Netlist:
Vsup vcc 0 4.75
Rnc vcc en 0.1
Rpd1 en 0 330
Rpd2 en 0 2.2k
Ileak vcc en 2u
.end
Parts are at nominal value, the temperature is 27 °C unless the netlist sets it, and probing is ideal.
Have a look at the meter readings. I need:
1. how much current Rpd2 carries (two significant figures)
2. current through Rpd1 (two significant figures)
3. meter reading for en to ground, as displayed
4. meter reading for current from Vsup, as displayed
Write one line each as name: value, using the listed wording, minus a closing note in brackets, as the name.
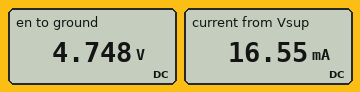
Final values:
how much current Rpd2 carries: 2.2 mA
current through Rpd1: 14 mA
meter reading for en to ground, as displayed: 4.748 V
meter reading for current from Vsup, as displayed: 16.55 mA
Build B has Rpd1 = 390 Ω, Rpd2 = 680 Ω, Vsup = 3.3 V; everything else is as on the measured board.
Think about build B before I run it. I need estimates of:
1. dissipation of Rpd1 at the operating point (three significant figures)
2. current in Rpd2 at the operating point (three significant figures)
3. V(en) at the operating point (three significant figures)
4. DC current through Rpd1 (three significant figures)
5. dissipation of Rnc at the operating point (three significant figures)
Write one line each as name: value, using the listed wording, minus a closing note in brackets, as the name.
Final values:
dissipation of Rpd1 at the operating point: 27.9 mW
current in Rpd2 at the operating point: 4.85 mA
V(en) at the operating point: 3.30 V
DC current through Rpd1: 8.46 mA
dissipation of Rnc at the operating point: 17.7 µW
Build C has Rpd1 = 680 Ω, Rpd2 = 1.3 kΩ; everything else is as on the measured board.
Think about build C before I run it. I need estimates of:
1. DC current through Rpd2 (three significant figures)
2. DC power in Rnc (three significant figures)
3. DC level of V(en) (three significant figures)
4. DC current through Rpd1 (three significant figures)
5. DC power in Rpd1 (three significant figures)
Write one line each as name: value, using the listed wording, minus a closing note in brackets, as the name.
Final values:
DC current through Rpd2: 3.65 mA
DC power in Rnc: 11.3 µW
DC level of V(en): 4.75 V
DC current through Rpd1: 6.98 mA
DC power in Rpd1: 33.2 mW
